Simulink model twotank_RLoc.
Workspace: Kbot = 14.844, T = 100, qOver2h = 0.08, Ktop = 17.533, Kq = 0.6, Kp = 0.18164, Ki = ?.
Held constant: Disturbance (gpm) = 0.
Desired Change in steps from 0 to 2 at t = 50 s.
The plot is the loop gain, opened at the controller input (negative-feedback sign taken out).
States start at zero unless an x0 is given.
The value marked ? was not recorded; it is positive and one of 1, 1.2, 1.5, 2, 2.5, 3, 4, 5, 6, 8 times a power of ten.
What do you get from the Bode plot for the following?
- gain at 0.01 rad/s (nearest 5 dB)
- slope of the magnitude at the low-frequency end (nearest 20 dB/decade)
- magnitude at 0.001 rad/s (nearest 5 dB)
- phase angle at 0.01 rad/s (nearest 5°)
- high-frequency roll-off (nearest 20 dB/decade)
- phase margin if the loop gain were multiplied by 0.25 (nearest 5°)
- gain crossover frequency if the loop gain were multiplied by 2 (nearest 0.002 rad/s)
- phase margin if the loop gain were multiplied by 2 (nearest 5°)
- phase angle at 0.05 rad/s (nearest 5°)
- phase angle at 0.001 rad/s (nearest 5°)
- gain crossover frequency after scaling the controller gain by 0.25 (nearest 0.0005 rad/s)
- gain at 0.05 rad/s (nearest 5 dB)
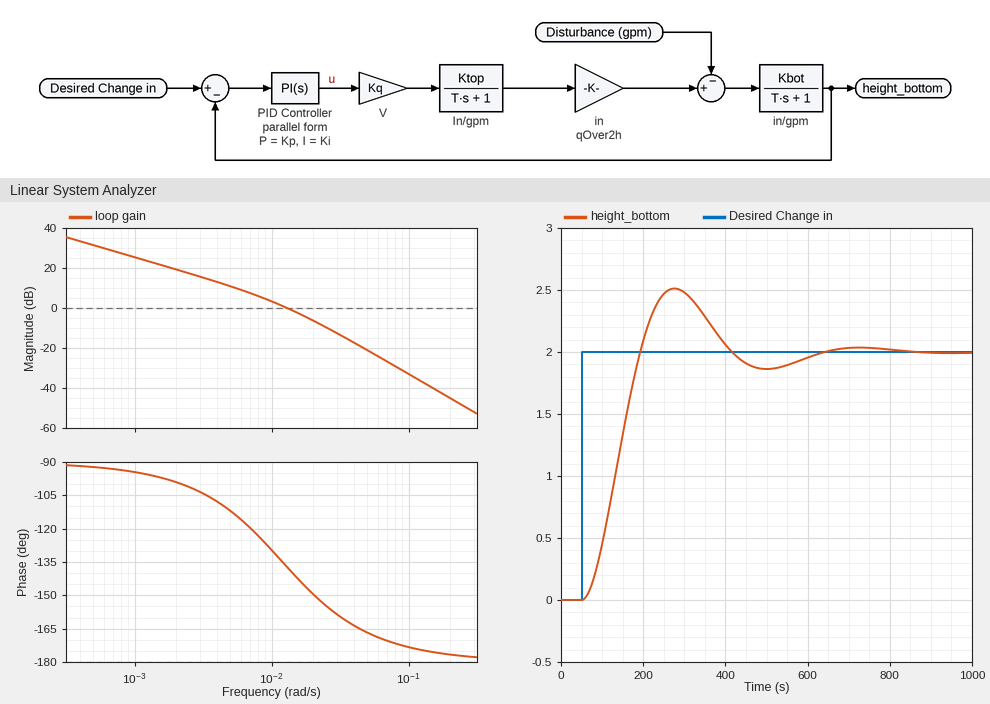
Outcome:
5 dB
-20 dB/decade
25 dB
-130°
-40 dB/decade
70°
0.020 rad/s
30°
-165°
-95°
0.0045 rad/s
-20 dB
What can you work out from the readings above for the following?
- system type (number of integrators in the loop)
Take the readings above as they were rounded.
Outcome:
1
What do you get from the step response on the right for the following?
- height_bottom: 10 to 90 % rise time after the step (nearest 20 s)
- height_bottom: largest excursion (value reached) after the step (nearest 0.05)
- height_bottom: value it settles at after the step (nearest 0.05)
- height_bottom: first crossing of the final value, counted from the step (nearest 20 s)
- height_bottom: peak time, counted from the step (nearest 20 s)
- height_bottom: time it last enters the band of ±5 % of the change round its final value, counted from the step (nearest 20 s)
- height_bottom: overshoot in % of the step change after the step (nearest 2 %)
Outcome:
100 s
2.50
2.00
140 s
220 s
500 s
26 %
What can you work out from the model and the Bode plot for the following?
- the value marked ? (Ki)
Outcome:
0.0015
